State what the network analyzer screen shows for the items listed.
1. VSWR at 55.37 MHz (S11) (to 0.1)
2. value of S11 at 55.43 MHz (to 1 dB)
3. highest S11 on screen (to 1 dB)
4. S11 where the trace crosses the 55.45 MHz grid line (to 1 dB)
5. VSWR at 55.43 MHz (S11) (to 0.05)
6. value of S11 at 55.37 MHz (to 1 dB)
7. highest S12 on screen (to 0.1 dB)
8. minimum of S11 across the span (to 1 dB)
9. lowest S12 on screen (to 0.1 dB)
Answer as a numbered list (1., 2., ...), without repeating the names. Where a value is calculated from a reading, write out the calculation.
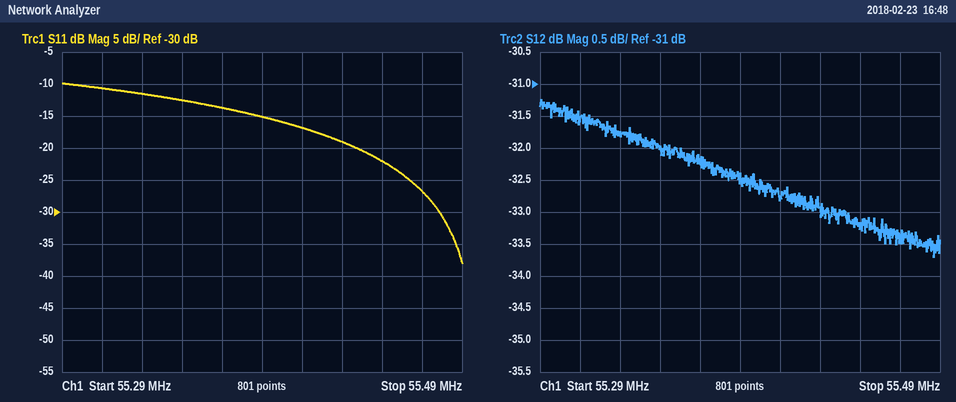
1. |Γ| = 10^(-14/20) = 0.1995; VSWR = (1 + 0.1995)/(1 − 0.1995) ≈ 1.5
2. -19 dB
3. -10 dB
4. -22 dB
5. |Γ| = 10^(-19/20) = 0.1122; VSWR = (1 + 0.1122)/(1 − 0.1122) ≈ 1.25
6. -14 dB
7. -31.2 dB
8. -38 dB
9. -33.7 dB
